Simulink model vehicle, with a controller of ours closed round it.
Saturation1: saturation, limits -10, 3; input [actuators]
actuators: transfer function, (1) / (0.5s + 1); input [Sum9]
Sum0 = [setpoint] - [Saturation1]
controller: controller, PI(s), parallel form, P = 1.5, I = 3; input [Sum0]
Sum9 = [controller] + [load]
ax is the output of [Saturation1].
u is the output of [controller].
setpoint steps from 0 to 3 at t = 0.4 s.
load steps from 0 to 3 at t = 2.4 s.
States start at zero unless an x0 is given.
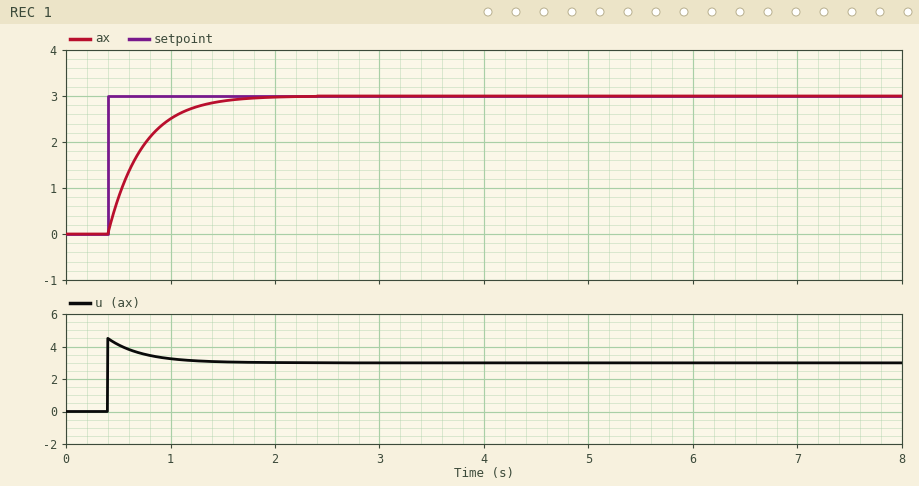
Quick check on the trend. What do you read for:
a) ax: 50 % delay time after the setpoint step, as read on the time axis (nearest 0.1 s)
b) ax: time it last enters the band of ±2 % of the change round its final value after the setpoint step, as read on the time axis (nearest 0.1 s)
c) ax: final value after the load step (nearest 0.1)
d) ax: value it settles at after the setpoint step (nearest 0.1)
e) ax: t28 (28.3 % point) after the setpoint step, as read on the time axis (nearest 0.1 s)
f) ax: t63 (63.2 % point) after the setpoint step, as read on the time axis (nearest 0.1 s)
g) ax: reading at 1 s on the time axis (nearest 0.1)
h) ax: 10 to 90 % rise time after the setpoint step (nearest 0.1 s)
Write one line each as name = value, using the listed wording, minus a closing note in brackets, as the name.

ax: 50 % delay time after the setpoint step, as read on the time axis = 0.6 s
ax: time it last enters the band of ±2 % of the change round its final value after the setpoint step, as read on the time axis = 1.7 s
ax: final value after the load step = 3.0
ax: value it settles at after the setpoint step = 3.0
ax: t28 (28.3 % point) after the setpoint step, as read on the time axis = 0.5 s
ax: t63 (63.2 % point) after the setpoint step, as read on the time axis = 0.7 s
ax: reading at 1 s on the time axis = 2.5
ax: 10 to 90 % rise time after the setpoint step = 0.7 s
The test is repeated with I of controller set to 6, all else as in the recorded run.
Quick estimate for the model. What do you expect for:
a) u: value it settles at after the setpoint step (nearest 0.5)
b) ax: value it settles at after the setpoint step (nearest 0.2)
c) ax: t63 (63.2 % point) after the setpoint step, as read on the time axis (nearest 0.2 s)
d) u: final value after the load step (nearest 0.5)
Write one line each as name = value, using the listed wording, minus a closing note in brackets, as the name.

u: value it settles at after the setpoint step = 4.0
ax: value it settles at after the setpoint step = 3.0
ax: t63 (63.2 % point) after the setpoint step, as read on the time axis = 0.6 s
u: final value after the load step = 4.0
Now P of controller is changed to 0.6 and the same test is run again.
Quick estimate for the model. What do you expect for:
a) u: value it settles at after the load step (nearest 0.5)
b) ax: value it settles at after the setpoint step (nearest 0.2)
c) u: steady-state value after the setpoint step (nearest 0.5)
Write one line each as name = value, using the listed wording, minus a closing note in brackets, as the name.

u: value it settles at after the load step = 3.5
ax: value it settles at after the setpoint step = 3.0
u: steady-state value after the setpoint step = 3.5
